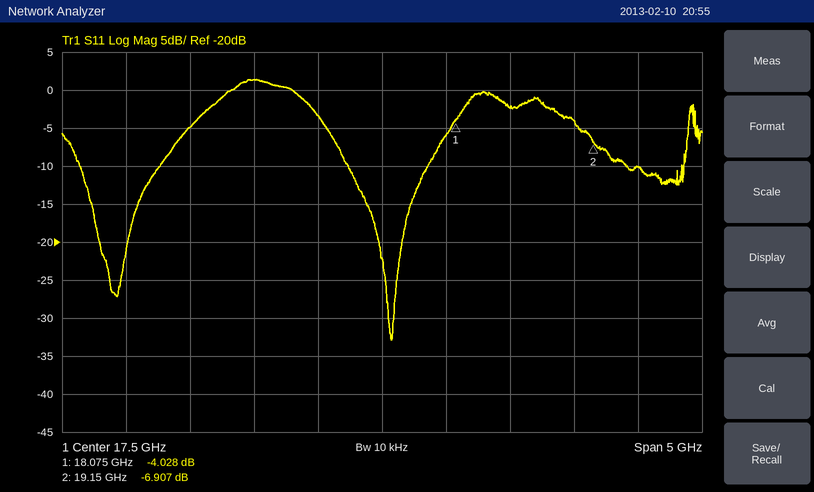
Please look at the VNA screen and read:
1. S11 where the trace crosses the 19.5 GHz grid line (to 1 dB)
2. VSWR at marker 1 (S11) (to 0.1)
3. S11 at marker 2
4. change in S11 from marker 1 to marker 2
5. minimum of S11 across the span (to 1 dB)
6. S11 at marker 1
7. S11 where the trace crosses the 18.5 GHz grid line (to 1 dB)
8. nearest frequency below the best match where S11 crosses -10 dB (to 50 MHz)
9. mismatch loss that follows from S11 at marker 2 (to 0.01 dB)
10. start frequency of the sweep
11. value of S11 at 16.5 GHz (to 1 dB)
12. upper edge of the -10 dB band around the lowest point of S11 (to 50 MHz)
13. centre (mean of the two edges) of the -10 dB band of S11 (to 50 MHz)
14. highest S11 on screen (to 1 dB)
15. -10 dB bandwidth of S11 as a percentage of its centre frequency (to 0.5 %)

-10 dB
4.4
-6.907 dB
-2.879 dB
-33 dB
-4.028 dB
-2 dB
17.25 GHz
0.99 dB
15 GHz
1 dB
17.85 GHz
17.55 GHz
1 dB
3.5 %
